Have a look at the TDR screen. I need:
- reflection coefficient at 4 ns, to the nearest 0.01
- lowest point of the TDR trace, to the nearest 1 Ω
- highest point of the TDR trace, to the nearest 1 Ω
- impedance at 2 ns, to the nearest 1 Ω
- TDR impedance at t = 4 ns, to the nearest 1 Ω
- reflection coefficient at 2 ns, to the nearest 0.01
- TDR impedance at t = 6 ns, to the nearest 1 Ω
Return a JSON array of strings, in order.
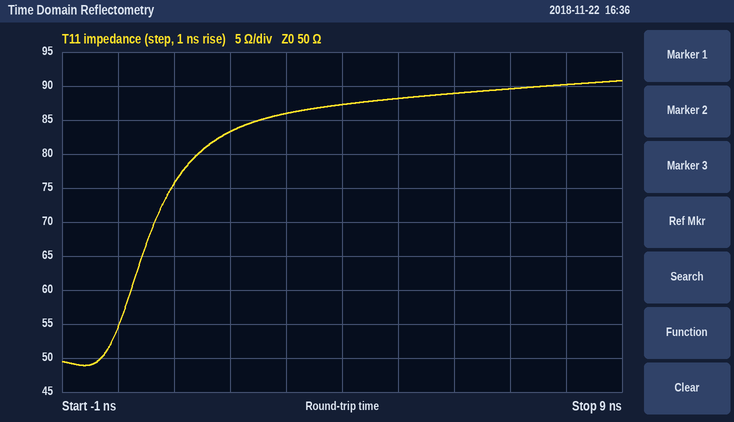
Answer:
["+0.27", "49 Ω", "91 Ω", "83 Ω", "87 Ω", "+0.25", "89 Ω"]
